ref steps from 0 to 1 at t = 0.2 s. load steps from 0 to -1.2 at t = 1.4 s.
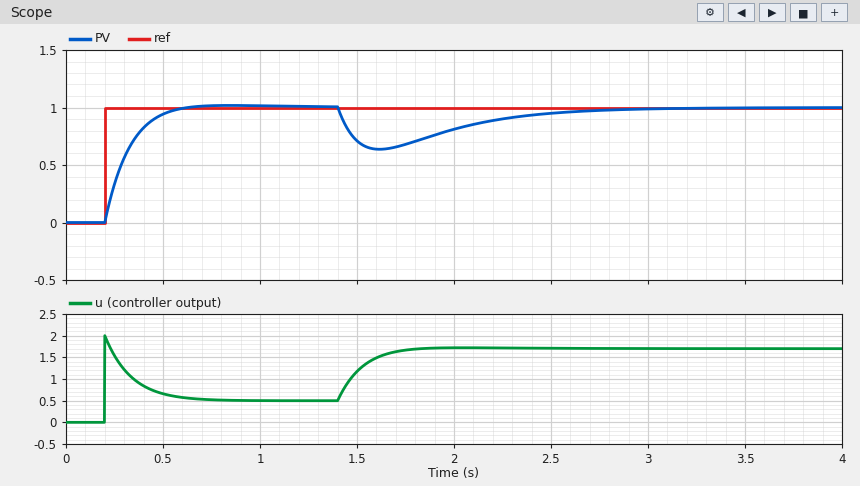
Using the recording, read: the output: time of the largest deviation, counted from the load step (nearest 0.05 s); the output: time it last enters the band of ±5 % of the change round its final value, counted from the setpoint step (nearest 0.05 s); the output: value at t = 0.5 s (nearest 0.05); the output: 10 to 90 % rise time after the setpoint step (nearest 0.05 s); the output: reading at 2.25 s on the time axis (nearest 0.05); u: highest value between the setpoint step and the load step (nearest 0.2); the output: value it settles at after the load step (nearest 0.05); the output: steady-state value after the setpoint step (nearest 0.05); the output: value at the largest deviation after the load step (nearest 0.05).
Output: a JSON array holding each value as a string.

["0.20 s", "0.30 s", "0.95", "0.25 s", "0.90", "2.0", "1.00", "1.00", "0.65"]
